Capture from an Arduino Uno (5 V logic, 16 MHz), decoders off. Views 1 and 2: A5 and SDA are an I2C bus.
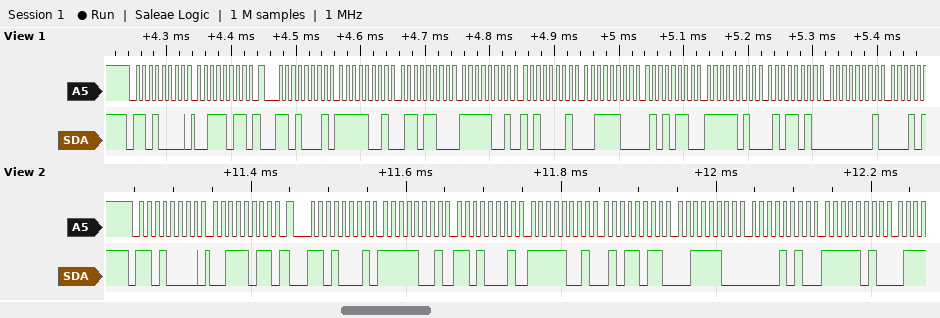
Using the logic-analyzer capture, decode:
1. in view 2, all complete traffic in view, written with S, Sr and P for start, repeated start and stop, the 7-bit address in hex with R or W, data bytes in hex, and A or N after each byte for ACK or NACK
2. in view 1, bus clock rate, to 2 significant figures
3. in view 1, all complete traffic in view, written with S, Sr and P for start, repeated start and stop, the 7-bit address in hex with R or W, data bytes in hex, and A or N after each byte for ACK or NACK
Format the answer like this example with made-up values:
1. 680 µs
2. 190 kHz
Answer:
1. S 68W A 3B A Sr 68R A F9 A D1 A F9 A 5B A 3C A 0A A FA A
2. 100 kHz
3. S 68W A 3B A Sr 68R A F9 A 6C A F9 A A1 A 3C A 56 A FA A 5A A 01 A
